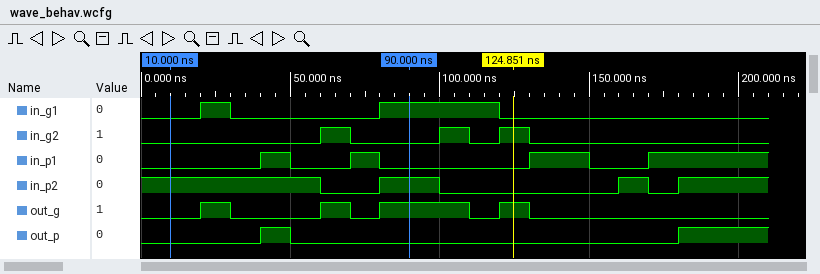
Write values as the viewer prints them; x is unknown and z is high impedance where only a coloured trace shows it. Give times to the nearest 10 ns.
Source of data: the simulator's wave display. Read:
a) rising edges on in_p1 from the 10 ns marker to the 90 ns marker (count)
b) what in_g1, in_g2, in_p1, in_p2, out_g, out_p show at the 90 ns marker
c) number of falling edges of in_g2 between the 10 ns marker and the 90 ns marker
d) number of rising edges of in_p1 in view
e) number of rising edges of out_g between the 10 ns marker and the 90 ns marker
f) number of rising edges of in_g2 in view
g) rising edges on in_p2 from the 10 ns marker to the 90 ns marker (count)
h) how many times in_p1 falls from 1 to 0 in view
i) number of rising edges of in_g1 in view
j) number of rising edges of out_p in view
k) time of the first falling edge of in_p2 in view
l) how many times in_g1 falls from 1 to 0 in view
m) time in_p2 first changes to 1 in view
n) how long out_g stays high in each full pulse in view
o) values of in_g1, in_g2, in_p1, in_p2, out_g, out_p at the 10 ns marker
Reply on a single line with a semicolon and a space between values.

2; in_g1=1, in_g2=0, in_p1=0, in_p2=1, out_g=1, out_p=0; 1; 4; 3; 3; 1; 3; 2; 2; 60 ns; 2; 80 ns; 10 ns, 10 ns, 30 ns, 10 ns; in_g1=0, in_g2=0, in_p1=0, in_p2=1, out_g=0, out_p=0
